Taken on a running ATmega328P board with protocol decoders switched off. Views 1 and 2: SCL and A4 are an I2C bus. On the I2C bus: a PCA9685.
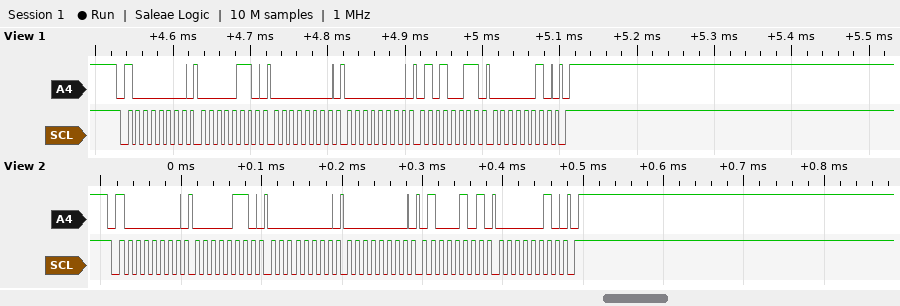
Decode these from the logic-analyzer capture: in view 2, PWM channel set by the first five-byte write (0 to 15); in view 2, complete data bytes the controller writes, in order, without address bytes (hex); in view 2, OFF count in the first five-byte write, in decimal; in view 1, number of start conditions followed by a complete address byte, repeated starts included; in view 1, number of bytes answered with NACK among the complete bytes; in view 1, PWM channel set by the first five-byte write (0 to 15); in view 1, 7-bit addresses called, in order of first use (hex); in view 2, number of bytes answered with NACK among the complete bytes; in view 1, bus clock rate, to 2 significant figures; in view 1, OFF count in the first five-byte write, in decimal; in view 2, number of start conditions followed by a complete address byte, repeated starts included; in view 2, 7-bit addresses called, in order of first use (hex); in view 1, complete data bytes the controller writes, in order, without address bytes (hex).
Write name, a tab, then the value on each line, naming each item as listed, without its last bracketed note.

in view 2, PWM channel set by the first five-byte write	0
in view 2, complete data bytes the controller writes, in order, without address bytes	06 00 00 45 02
in view 2, OFF count in the first five-byte write, in decimal	581
in view 1, number of start conditions followed by a complete address byte, repeated starts included	1
in view 1, number of bytes answered with NACK among the complete bytes	0
in view 1, PWM channel set by the first five-byte write	0
in view 1, 7-bit addresses called, in order of first use	0x40
in view 2, number of bytes answered with NACK among the complete bytes	0
in view 1, bus clock rate, to 2 significant figures	100 kHz
in view 1, OFF count in the first five-byte write, in decimal	595
in view 2, number of start conditions followed by a complete address byte, repeated starts included	1
in view 2, 7-bit addresses called, in order of first use	0x40
in view 1, complete data bytes the controller writes, in order, without address bytes	06 00 00 53 02
